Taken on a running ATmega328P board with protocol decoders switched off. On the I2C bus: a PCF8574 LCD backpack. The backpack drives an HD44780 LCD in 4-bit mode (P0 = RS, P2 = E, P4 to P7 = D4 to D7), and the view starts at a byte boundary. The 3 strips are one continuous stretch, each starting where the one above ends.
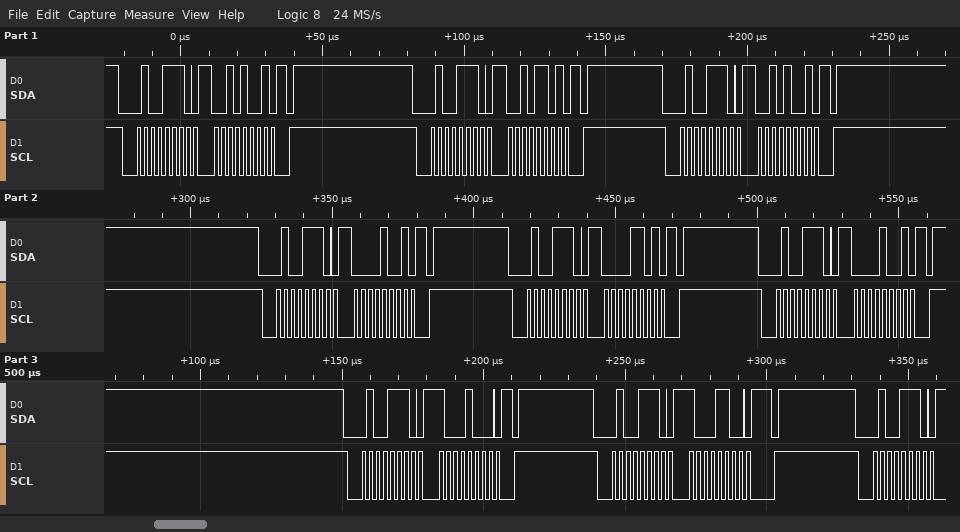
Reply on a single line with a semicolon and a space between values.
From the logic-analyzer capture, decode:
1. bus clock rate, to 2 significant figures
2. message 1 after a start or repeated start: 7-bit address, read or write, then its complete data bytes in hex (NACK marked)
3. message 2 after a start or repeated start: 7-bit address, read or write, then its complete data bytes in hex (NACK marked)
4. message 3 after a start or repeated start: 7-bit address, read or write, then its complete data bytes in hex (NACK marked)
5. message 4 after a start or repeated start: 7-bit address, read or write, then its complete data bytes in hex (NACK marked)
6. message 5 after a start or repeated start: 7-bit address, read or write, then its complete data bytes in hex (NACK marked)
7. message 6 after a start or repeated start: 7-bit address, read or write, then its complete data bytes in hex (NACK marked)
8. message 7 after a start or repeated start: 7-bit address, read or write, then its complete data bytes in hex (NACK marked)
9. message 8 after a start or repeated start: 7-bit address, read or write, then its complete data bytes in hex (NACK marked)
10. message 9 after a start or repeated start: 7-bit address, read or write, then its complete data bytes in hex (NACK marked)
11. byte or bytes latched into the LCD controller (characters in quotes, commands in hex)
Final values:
400 kHz; 0x27 write: 29; 0x27 write: 2D; 0x27 write: 29; 0x27 write: 09; 0x27 write: 0D; 0x27 write: 09; 0x27 write: 88; 0x27 write: 8C; 0x27 write; ' '
